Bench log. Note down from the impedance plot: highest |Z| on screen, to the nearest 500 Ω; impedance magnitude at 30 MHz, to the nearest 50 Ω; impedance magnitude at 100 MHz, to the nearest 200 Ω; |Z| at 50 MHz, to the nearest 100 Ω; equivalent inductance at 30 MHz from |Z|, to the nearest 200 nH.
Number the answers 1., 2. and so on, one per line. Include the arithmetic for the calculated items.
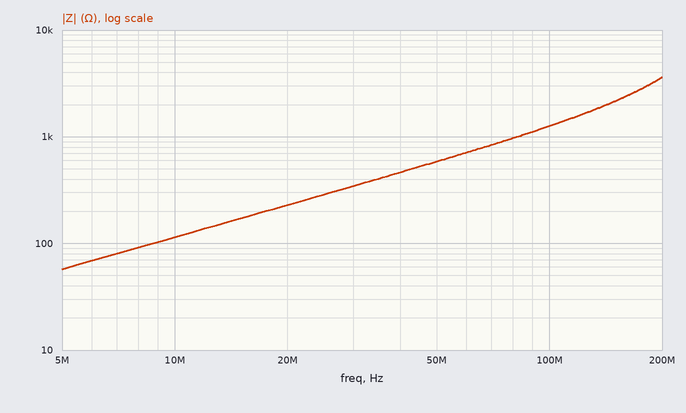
1. 3.5 kΩ
2. 350 Ω
3. 1.2 kΩ
4. 600 Ω
5. L = 350 Ω/(2π × 30 MHz) ≈ 1.86 µH, so 1.8 µH to the nearest 200 nH
